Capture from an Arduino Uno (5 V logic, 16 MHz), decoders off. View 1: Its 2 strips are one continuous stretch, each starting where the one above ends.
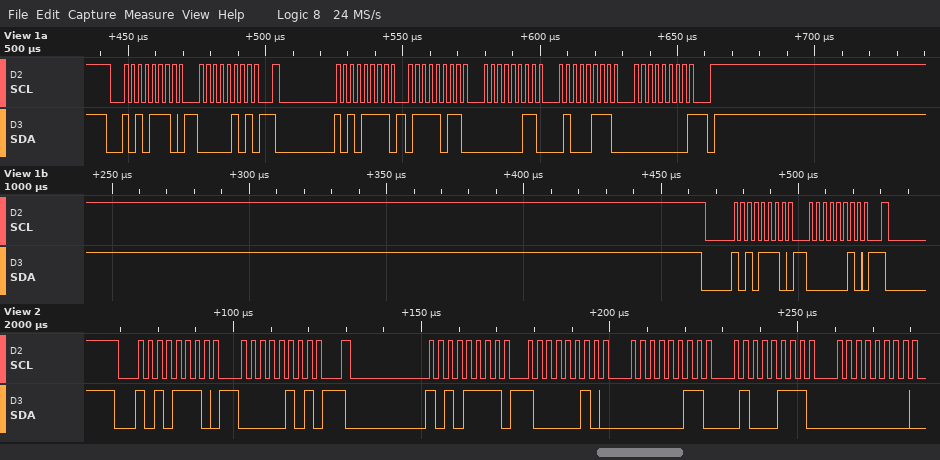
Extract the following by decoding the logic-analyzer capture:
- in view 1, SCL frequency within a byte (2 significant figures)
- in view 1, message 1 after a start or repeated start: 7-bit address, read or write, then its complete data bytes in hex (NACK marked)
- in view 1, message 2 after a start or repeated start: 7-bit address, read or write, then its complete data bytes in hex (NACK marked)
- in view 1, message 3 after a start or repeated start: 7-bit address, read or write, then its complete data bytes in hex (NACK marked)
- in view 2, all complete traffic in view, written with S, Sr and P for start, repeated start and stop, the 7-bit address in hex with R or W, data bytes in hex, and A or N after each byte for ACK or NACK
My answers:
400 kHz
0x57 write: 05
0x57 read: 7B 03 47 00 NACK
0x57 write: 02
S 57W A 05 A Sr 57R A 82 A 03 A 47 A 00 A
